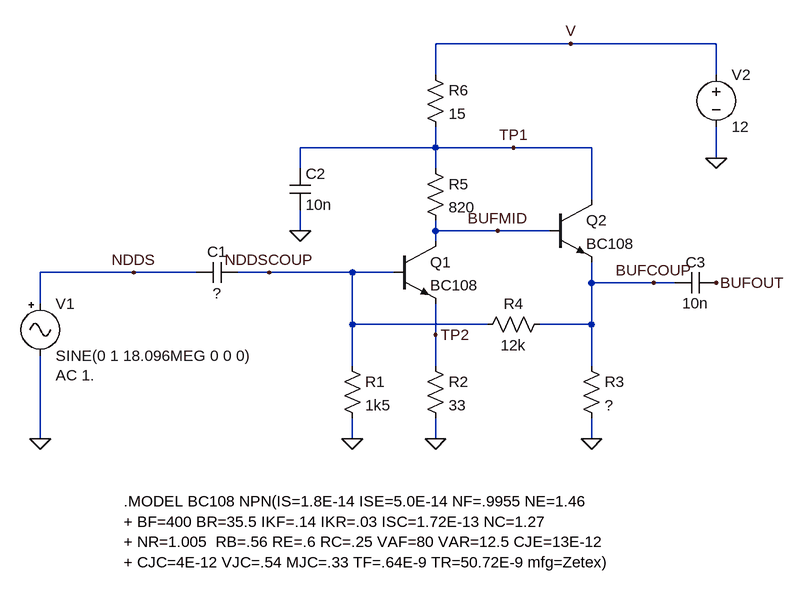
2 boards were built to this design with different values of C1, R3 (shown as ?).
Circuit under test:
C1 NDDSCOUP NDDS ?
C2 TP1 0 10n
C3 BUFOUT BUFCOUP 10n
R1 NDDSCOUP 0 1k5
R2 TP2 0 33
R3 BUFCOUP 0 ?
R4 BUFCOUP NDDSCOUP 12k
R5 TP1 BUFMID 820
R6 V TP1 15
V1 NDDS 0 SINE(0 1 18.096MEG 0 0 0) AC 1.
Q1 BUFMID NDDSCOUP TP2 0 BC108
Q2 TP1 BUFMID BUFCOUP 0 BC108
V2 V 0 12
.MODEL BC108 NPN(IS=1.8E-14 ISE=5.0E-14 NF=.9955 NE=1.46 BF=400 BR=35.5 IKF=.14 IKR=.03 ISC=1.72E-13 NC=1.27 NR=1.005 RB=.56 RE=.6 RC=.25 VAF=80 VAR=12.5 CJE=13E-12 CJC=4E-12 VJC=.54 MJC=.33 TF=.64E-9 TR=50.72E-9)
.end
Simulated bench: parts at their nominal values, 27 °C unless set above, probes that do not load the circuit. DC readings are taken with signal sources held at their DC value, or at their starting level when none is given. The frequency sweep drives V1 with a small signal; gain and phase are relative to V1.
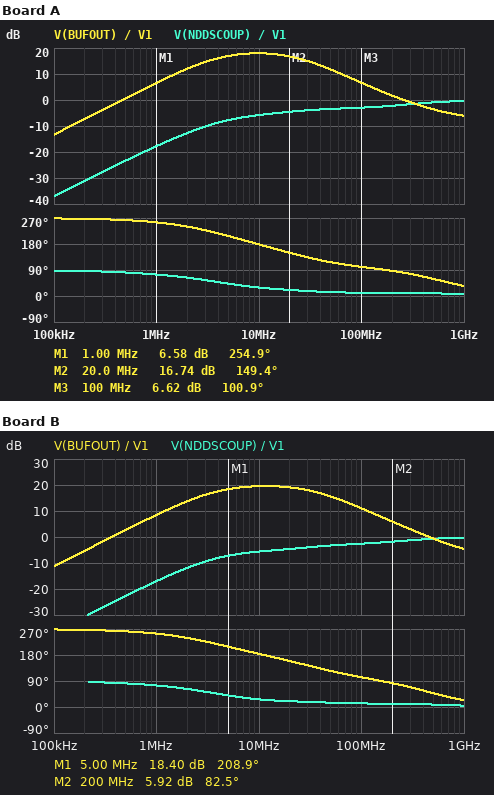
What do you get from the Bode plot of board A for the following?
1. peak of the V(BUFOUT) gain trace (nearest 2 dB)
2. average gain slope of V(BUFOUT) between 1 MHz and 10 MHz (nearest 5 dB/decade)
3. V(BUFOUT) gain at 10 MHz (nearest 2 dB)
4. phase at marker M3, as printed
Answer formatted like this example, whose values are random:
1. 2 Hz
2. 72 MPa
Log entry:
1. 18 dB
2. 10 dB/decade
3. 18 dB
4. 100.9 deg
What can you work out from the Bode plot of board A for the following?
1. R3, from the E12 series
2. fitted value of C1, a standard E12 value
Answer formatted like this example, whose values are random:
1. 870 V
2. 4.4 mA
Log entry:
1. 82 Ω
2. 47 pF
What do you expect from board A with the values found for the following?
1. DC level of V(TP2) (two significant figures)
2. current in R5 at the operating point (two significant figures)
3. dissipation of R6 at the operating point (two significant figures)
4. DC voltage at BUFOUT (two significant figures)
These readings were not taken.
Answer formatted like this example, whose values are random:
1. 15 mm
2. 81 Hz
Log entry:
1. 100 mV
2. 3.4 mA
3. 120 mW
4. 7.0 V
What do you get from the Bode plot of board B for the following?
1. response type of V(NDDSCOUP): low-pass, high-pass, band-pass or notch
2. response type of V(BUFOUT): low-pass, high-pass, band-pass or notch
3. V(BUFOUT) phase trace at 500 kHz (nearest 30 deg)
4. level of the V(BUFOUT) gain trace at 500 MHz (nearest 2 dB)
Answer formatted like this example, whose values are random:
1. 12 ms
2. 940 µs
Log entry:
1. high-pass
2. band-pass
3. 270 deg
4. 0 dB
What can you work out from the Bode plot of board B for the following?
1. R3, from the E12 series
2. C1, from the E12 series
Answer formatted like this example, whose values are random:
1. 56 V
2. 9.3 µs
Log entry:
1. 180 Ω
2. 56 pF
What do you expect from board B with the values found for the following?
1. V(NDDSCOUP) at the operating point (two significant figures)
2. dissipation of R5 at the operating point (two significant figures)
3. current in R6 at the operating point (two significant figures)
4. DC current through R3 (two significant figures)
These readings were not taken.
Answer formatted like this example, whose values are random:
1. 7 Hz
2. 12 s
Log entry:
1. 800 mV
2. 13 mW
3. 45 mA
4. 41 mA
